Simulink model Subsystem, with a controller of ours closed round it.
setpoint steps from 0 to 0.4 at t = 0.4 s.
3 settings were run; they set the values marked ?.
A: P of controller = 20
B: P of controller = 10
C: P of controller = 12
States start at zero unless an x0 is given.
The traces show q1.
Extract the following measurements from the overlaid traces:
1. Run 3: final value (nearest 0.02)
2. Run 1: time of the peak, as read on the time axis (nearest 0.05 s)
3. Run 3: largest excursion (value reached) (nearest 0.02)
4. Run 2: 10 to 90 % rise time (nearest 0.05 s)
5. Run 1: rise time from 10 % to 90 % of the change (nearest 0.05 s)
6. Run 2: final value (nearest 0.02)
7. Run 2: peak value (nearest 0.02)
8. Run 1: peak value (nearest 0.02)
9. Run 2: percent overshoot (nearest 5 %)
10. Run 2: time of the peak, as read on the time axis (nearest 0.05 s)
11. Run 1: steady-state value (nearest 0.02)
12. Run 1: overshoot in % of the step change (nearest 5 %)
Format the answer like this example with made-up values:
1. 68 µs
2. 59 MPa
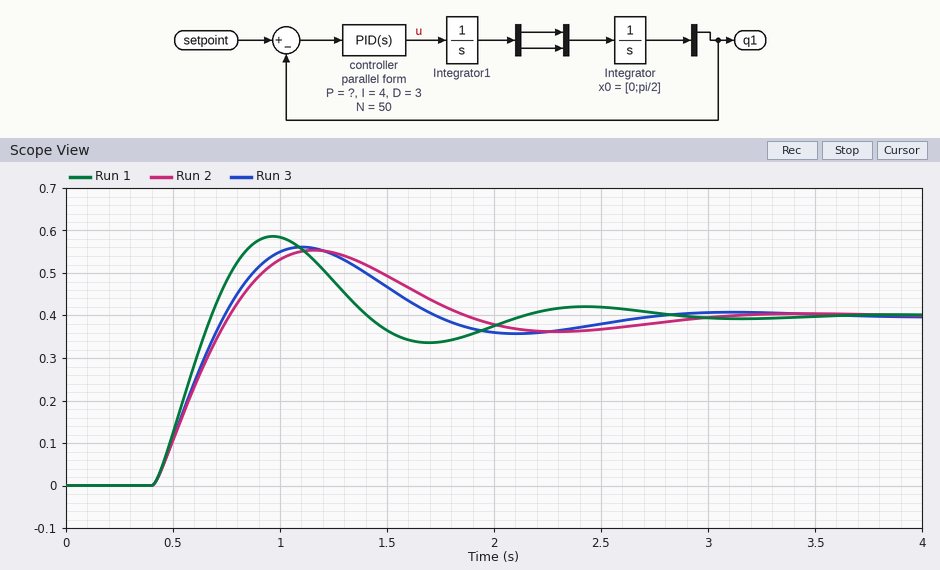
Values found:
1. 0.40
2. 0.95 s
3. 0.56
4. 0.25 s
5. 0.20 s
6. 0.40
7. 0.56
8. 0.58
9. 40 %
10. 1.15 s
11. 0.40
12. 45 %
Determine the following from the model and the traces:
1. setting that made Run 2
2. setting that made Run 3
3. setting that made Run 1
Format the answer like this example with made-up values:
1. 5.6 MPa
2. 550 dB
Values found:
1. B
2. C
3. A
